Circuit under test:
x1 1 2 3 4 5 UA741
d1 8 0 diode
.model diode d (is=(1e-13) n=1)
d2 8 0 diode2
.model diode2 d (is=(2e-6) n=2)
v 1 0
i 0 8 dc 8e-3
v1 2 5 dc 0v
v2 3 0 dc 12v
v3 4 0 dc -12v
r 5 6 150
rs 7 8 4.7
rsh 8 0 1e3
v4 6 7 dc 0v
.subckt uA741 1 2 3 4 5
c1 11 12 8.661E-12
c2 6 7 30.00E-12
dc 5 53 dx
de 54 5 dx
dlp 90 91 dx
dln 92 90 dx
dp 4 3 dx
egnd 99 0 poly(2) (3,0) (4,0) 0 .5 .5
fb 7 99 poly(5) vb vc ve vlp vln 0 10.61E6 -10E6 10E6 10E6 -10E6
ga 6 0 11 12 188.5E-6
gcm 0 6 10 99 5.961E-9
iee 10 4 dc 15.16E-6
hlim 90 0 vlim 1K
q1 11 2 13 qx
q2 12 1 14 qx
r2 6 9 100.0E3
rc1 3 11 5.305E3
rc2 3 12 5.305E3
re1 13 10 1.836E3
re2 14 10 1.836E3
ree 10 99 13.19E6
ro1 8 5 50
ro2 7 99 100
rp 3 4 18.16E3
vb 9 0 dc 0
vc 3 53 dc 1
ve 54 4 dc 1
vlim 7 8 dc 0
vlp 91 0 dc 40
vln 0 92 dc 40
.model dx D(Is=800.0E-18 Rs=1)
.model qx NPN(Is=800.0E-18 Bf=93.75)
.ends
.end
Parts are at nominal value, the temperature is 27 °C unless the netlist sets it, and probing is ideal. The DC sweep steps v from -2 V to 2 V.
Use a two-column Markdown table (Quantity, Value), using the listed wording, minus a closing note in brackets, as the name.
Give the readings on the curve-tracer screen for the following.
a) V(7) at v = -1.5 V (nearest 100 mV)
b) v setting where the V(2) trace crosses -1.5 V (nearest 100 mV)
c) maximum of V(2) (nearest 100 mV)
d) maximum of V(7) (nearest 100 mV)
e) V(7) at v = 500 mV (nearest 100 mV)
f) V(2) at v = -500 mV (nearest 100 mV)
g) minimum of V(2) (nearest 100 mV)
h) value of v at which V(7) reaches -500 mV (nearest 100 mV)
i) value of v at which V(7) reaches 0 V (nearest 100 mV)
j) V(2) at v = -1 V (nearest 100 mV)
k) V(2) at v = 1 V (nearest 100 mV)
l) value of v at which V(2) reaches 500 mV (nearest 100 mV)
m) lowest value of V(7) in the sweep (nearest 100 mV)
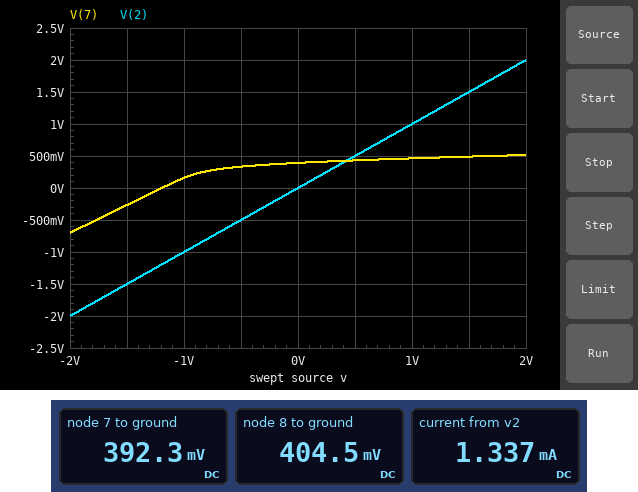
| Quantity | Value |
|---|---|
| V(7) at v = -1.5 V | -300 mV |
| v setting where the V(2) trace crosses -1.5 V | -1.5 V |
| maximum of V(2) | 2.0 V |
| maximum of V(7) | 500 mV |
| V(7) at v = 500 mV | 400 mV |
| V(2) at v = -500 mV | -500 mV |
| minimum of V(2) | -2.0 V |
| value of v at which V(7) reaches -500 mV | -1.8 V |
| value of v at which V(7) reaches 0 V | -1.2 V |
| V(2) at v = -1 V | -1.0 V |
| V(2) at v = 1 V | 1.0 V |
| value of v at which V(2) reaches 500 mV | 500 mV |
| lowest value of V(7) in the sweep | -700 mV |
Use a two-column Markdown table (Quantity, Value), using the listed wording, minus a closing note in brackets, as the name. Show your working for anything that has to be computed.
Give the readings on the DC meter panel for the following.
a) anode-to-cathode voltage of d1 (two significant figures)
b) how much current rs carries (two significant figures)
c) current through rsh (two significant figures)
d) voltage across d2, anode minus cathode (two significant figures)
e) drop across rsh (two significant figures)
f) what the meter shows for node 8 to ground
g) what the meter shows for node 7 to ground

| Quantity | Value |
|---|---|
| anode-to-cathode voltage of d1 | 404.5 mV = 400 mV |
| how much current rs carries | (404.5 mV - 392.3 mV) / 4.7 Ω = 2.6 mA |
| current through rsh | (404.5 mV) / 1 kΩ = 400 µA |
| voltage across d2, anode minus cathode | 404.5 mV = 400 mV |
| drop across rsh | 404.5 mV = 400 mV |
| what the meter shows for node 8 to ground | 404.5 mV |
| what the meter shows for node 7 to ground | 392.3 mV |
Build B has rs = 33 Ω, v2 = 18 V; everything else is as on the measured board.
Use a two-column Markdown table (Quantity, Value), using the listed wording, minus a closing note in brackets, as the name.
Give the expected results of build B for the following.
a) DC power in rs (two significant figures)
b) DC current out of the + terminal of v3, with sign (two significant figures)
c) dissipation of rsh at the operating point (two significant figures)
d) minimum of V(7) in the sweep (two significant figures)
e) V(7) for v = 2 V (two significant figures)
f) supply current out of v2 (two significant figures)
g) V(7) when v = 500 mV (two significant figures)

| Quantity | Value |
|---|---|
| DC power in rs | 160 µW |
| DC current out of the + terminal of v3, with sign | -1.7 mA |
| dissipation of rsh at the operating point | 170 µW |
| minimum of V(7) in the sweep | -730 mV |
| V(7) for v = 2 V | 740 mV |
| supply current out of v2 | 1.7 mA |
| V(7) when v = 500 mV | 440 mV |
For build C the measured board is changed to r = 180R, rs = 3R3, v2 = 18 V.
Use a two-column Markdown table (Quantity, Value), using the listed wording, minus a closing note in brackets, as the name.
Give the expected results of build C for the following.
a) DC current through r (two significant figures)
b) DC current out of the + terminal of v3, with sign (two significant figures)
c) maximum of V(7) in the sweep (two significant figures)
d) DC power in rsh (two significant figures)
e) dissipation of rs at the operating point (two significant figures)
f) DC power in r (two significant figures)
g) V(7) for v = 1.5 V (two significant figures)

| Quantity | Value |
|---|---|
| DC current through r | 2.2 mA |
| DC current out of the + terminal of v3, with sign | -1.7 mA |
| maximum of V(7) in the sweep | 490 mV |
| DC power in rsh | 170 µW |
| dissipation of rs at the operating point | 16 µW |
| DC power in r | 890 µW |
| V(7) for v = 1.5 V | 470 mV |
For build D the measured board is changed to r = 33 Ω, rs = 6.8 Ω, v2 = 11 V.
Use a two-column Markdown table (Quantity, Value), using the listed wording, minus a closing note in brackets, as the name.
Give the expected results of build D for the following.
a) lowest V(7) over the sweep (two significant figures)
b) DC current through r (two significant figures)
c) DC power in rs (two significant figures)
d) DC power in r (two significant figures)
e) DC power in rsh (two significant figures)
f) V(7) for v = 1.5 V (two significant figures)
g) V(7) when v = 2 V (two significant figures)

| Quantity | Value |
|---|---|
| lowest V(7) over the sweep | -1.7 V |
| DC current through r | 7.2 mA |
| DC power in rs | 350 µW |
| DC power in r | 1.7 mW |
| DC power in rsh | 82 µW |
| V(7) for v = 1.5 V | 670 mV |
| V(7) when v = 2 V | 770 mV |
